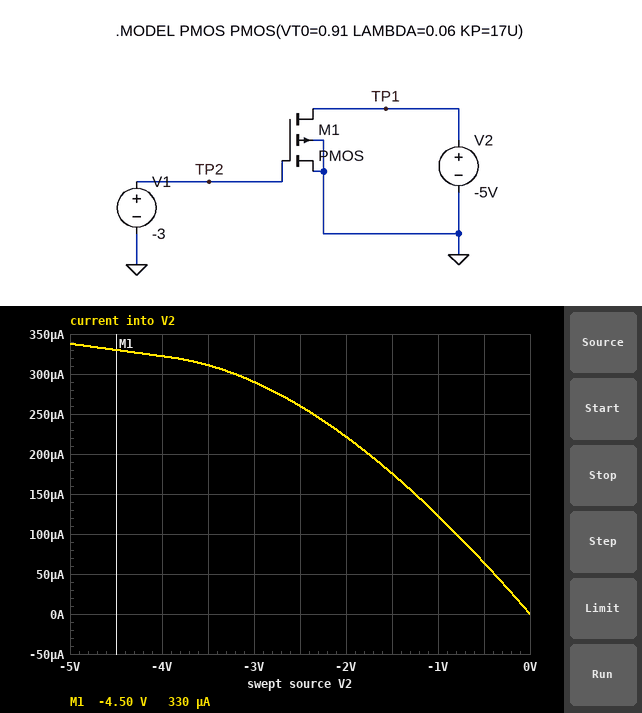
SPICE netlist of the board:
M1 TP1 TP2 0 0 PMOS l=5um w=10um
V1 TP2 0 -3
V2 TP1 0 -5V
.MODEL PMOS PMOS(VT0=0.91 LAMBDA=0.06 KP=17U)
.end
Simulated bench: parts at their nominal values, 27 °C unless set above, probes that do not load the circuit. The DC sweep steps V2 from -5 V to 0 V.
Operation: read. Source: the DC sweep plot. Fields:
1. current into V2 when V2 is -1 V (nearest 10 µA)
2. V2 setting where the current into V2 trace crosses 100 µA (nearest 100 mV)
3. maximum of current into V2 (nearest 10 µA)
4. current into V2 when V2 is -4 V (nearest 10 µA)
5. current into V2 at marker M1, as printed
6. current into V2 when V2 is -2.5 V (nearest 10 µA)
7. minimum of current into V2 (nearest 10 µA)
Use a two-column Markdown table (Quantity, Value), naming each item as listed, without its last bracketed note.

| Quantity | Value |
|---|---|
| current into V2 when V2 is -1 V | 120 µA |
| V2 setting where the current into V2 trace crosses 100 µA | -800 mV |
| maximum of current into V2 | 340 µA |
| current into V2 when V2 is -4 V | 320 µA |
| current into V2 at marker M1, as printed | 330 µA |
| current into V2 when V2 is -2.5 V | 260 µA |
| minimum of current into V2 | 0 A |
